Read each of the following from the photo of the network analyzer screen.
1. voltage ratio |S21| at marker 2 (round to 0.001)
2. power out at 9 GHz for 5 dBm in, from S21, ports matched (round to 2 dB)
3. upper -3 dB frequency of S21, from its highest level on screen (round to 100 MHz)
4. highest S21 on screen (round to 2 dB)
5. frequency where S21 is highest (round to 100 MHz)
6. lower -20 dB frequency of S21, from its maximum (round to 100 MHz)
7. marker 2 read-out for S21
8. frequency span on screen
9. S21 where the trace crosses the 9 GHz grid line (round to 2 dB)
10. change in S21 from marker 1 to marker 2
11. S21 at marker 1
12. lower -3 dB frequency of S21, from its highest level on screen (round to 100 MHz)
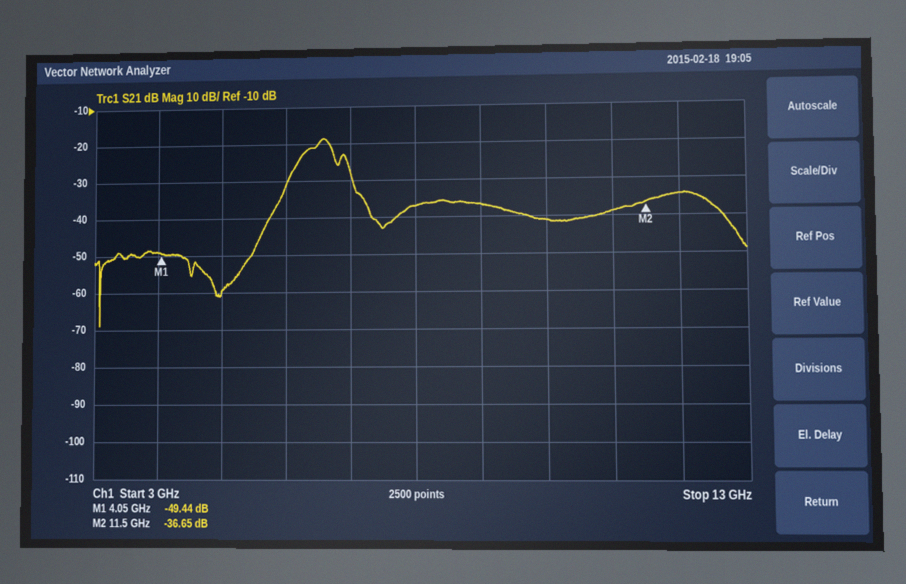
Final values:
0.015
-32 dBm
6.7 GHz
-18 dB
6.6 GHz
5.8 GHz
-36.65 dB
10 GHz
-36 dB
12.79 dB
-49.44 dB
6.3 GHz
